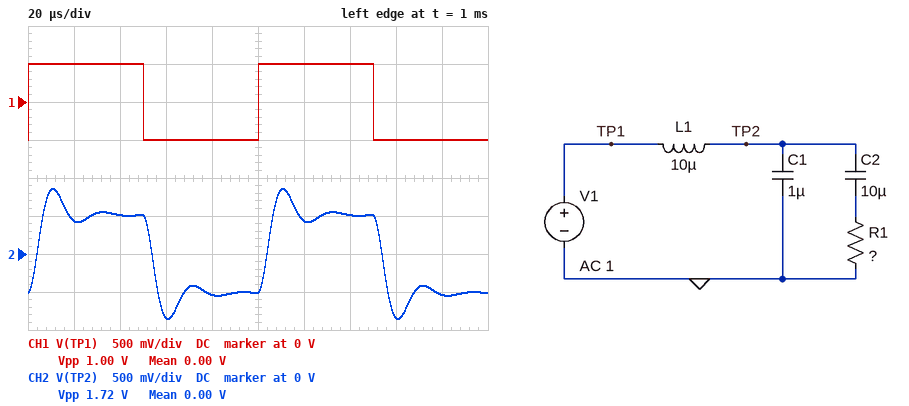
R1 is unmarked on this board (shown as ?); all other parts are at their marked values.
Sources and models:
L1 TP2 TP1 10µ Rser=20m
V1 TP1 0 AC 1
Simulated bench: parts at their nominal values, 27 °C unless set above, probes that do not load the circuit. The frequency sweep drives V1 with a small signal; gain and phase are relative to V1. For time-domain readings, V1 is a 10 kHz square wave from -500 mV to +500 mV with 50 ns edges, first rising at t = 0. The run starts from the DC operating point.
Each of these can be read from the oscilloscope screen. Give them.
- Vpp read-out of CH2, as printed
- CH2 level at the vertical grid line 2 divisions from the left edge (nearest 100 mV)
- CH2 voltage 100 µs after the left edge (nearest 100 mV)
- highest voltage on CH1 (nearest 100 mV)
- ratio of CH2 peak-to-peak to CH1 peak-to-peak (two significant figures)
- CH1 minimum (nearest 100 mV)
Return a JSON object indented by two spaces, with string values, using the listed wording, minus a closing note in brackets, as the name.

{
  "Vpp read-out of CH2, as printed": "1.72 V",
  "CH2 level at the vertical grid line 2 divisions from the left edge": "500 mV",
  "CH2 voltage 100 µs after the left edge": "-500 mV",
  "highest voltage on CH1": "500 mV",
  "ratio of CH2 peak-to-peak to CH1 peak-to-peak": "1.7",
  "CH1 minimum": "-500 mV"
}
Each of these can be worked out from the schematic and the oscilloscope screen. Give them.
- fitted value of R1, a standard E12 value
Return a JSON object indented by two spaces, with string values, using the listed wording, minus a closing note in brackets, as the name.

{
  "fitted value of R1, a standard E12 value": "4.7 Ω"
}
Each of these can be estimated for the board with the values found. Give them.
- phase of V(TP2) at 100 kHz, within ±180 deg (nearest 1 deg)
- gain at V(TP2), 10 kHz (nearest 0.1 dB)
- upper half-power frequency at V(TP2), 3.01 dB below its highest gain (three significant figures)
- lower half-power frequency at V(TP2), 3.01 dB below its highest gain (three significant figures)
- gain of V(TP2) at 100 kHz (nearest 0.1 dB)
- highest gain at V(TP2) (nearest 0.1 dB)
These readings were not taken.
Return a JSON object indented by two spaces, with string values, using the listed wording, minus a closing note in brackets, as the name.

{
  "phase of V(TP2) at 100 kHz, within ±180 deg": "-156 deg",
  "gain at V(TP2), 10 kHz": "0.6 dB",
  "upper half-power frequency at V(TP2), 3.01 dB below its highest gain": "58.5 kHz",
  "lower half-power frequency at V(TP2), 3.01 dB below its highest gain": "16.7 kHz",
  "gain of V(TP2) at 100 kHz": "-10.3 dB",
  "highest gain at V(TP2)": "4.1 dB"
}
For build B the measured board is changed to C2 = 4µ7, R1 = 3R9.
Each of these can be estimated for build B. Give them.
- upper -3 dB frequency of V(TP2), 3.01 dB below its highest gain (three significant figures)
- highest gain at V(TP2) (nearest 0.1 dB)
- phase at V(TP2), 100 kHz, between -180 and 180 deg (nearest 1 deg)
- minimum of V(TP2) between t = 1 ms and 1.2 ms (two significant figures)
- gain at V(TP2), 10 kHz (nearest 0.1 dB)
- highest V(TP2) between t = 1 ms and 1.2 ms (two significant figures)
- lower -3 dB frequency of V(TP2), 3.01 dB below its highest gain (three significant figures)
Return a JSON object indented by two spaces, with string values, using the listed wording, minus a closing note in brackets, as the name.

{
  "upper -3 dB frequency of V(TP2), 3.01 dB below its highest gain": "55.1 kHz",
  "highest gain at V(TP2)": "3.6 dB",
  "phase at V(TP2), 100 kHz, between -180 and 180 deg": "-152 deg",
  "minimum of V(TP2) between t = 1 ms and 1.2 ms": "-870 mV",
  "gain at V(TP2), 10 kHz": "1.0 dB",
  "highest V(TP2) between t = 1 ms and 1.2 ms": "870 mV",
  "lower -3 dB frequency of V(TP2), 3.01 dB below its highest gain": "6.65 kHz"
}
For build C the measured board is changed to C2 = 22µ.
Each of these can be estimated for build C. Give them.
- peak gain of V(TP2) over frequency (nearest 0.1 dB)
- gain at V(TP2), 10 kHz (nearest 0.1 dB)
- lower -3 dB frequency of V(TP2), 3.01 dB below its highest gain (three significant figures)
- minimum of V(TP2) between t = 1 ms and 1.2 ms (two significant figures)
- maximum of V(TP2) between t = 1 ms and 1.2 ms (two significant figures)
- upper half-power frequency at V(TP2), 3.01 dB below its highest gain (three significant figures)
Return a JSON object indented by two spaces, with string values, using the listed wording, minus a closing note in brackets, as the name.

{
  "peak gain of V(TP2) over frequency": "4.0 dB",
  "gain at V(TP2), 10 kHz": "0.4 dB",
  "lower -3 dB frequency of V(TP2), 3.01 dB below its highest gain": "17.5 kHz",
  "minimum of V(TP2) between t = 1 ms and 1.2 ms": "-830 mV",
  "maximum of V(TP2) between t = 1 ms and 1.2 ms": "830 mV",
  "upper half-power frequency at V(TP2), 3.01 dB below its highest gain": "59.2 kHz"
}
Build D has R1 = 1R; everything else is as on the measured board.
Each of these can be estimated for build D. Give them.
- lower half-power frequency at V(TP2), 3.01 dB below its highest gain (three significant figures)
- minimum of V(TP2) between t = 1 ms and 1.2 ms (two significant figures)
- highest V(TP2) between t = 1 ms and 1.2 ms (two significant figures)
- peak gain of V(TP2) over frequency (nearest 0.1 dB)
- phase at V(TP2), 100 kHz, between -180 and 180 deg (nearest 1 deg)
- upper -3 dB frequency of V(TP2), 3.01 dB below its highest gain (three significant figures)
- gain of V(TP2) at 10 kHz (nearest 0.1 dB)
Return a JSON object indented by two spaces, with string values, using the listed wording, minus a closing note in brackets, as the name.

{
  "lower half-power frequency at V(TP2), 3.01 dB below its highest gain": "5.19 kHz",
  "minimum of V(TP2) between t = 1 ms and 1.2 ms": "-870 mV",
  "highest V(TP2) between t = 1 ms and 1.2 ms": "870 mV",
  "peak gain of V(TP2) over frequency": "4.0 dB",
  "phase at V(TP2), 100 kHz, between -180 and 180 deg": "-122 deg",
  "upper -3 dB frequency of V(TP2), 3.01 dB below its highest gain": "21.4 kHz",
  "gain of V(TP2) at 10 kHz": "3.0 dB"
}
